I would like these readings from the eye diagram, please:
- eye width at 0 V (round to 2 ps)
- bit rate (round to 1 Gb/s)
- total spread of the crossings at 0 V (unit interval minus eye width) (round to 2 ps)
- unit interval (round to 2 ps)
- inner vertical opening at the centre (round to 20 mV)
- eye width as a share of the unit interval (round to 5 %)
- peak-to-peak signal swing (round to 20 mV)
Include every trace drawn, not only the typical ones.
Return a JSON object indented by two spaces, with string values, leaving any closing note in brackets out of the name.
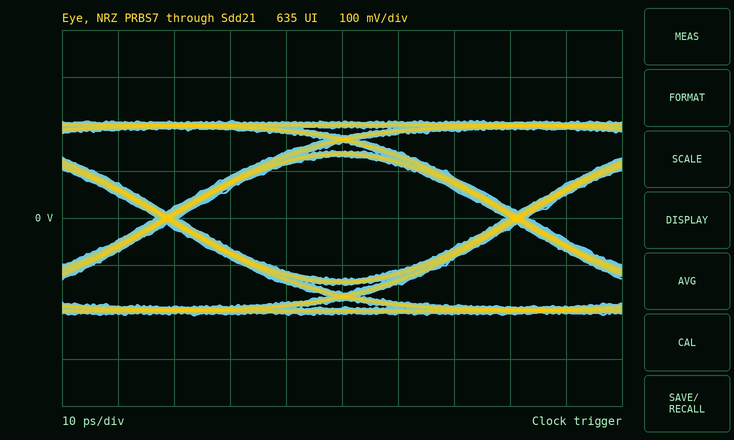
{
  "eye width at 0 V": "58 ps",
  "bit rate": "16 Gb/s",
  "total spread of the crossings at 0 V (unit interval minus eye width)": "4 ps",
  "unit interval": "62 ps",
  "inner vertical opening at the centre": "260 mV",
  "eye width as a share of the unit interval": "95 %",
  "peak-to-peak signal swing": "420 mV"
}
